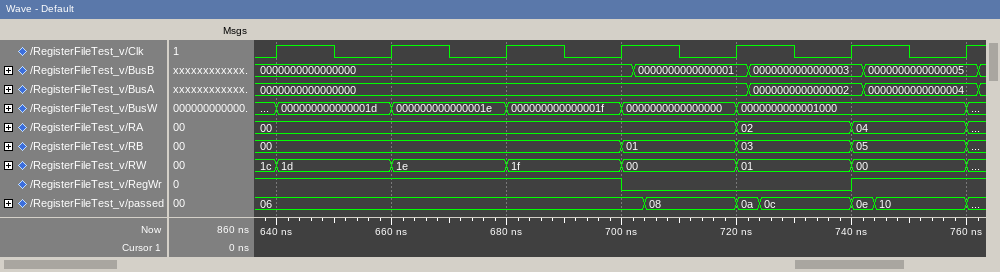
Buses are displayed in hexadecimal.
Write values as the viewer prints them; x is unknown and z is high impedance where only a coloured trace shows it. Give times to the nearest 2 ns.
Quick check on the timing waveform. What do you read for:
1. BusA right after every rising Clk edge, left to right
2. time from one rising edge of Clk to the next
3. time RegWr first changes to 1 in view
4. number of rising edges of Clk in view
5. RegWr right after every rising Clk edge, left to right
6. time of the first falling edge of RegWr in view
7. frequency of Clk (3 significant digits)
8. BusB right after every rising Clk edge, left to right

0000000000000000, 0000000000000000, 0000000000000000, 0000000000000000, 0000000000000000, 0000000000000002, 0000000000000004
20 ns
740 ns
7
1 1 1 0 0 1 1
700 ns
50.0 MHz
0000000000000000, 0000000000000000, 0000000000000000, 0000000000000000, 0000000000000001, 0000000000000003, 0000000000000005
